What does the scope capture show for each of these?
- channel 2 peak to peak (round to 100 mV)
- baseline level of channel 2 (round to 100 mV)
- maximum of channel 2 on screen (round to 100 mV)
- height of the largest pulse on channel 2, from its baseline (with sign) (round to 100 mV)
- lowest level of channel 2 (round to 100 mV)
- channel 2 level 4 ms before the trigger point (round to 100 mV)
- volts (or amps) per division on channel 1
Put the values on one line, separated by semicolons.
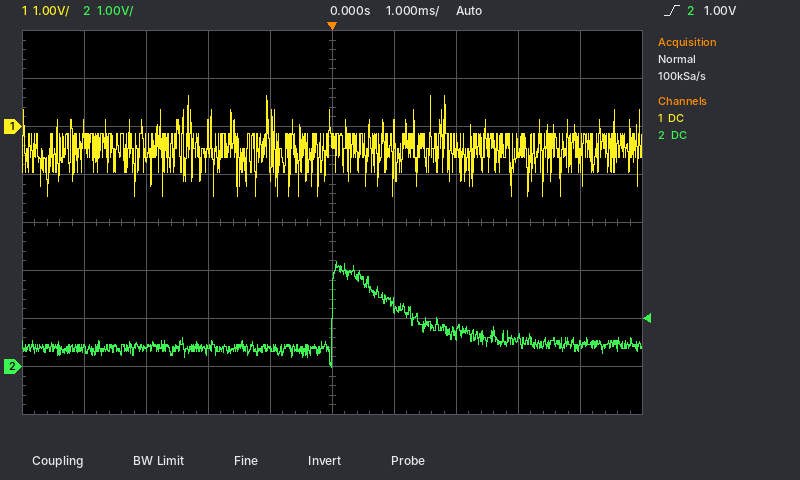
2.2 V; 400 mV; 2.2 V; +1.8 V; 0.0 V; 400 mV; 1 V
